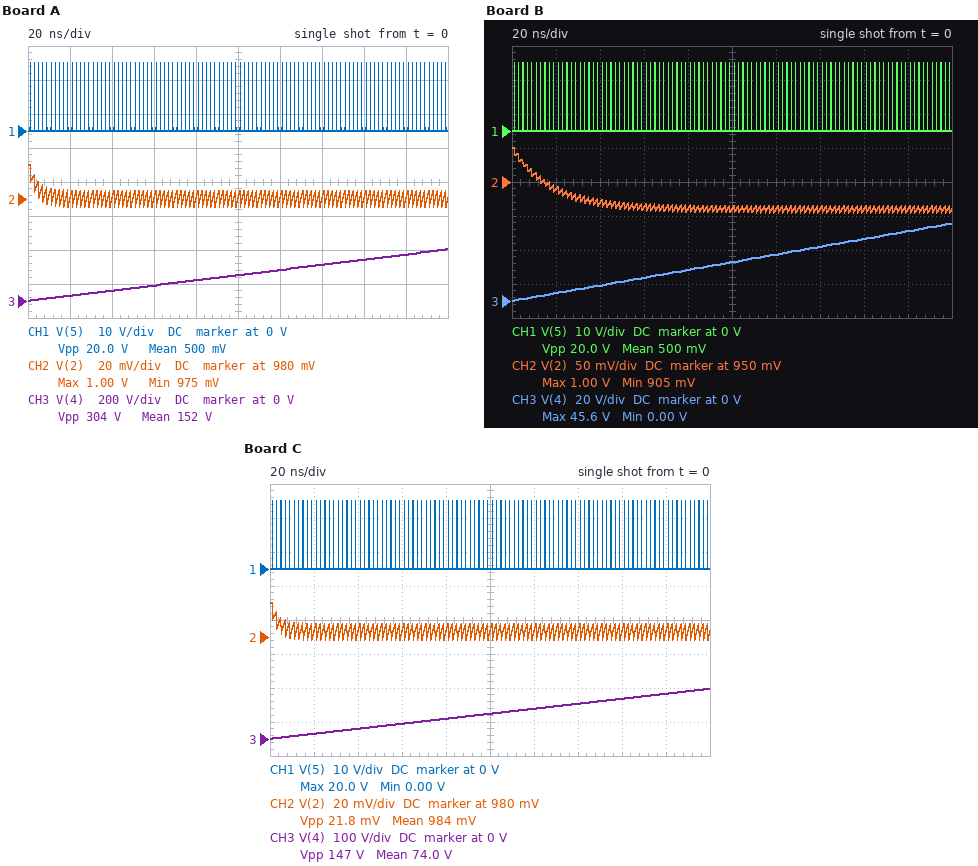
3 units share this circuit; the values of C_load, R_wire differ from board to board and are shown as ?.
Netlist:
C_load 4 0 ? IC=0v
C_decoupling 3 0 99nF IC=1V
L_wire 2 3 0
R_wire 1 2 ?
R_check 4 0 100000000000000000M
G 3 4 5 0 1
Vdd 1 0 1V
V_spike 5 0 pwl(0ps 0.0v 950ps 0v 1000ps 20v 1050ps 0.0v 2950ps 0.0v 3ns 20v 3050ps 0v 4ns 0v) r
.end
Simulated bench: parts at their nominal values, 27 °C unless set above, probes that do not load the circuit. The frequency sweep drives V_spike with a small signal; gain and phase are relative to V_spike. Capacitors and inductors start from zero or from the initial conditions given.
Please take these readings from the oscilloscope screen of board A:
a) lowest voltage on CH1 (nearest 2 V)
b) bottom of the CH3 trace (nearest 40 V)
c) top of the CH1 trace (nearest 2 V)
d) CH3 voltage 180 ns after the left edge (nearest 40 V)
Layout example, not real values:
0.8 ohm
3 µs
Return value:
0 V
0 V
20 V
280 V
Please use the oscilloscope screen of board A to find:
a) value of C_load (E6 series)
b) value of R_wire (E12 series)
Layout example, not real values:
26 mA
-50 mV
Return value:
330 pF
0.039 Ω
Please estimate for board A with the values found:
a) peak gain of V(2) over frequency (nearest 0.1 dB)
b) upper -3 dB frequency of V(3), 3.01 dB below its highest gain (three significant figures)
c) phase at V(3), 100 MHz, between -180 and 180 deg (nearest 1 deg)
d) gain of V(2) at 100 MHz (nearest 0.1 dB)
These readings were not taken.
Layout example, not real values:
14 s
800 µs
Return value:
-28.2 dB
41.2 MHz
112 deg
-36.6 dB
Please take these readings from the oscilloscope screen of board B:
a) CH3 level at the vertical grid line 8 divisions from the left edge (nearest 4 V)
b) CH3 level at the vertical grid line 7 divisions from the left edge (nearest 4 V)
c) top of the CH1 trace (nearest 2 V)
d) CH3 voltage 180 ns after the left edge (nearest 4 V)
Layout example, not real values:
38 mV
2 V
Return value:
36 V
32 V
20 V
40 V
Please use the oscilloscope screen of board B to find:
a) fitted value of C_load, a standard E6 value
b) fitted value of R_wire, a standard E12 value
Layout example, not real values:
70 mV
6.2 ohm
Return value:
2.2 nF
0.18 Ω
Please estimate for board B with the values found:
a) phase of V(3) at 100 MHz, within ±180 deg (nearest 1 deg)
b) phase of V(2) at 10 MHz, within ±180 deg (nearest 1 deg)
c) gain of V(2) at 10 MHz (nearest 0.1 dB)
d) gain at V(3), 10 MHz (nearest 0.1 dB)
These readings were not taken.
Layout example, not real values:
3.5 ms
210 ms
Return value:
95 deg
132 deg
-18.4 dB
-18.4 dB
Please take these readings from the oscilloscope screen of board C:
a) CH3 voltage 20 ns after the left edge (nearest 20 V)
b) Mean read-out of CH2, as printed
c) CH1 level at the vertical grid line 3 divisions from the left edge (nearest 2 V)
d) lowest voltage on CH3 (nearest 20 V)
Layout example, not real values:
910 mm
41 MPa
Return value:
20 V
984 mV
0 V
0 V
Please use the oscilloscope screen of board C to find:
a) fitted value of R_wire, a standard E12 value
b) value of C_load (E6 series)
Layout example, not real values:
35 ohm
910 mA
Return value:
0.033 Ω
680 pF
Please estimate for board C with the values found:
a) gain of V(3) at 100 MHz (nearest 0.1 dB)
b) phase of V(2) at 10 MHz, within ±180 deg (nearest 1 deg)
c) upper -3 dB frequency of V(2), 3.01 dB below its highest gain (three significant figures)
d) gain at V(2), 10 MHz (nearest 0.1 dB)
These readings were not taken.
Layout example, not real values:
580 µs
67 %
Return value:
-36.8 dB
168 deg
48.7 MHz
-29.8 dB
